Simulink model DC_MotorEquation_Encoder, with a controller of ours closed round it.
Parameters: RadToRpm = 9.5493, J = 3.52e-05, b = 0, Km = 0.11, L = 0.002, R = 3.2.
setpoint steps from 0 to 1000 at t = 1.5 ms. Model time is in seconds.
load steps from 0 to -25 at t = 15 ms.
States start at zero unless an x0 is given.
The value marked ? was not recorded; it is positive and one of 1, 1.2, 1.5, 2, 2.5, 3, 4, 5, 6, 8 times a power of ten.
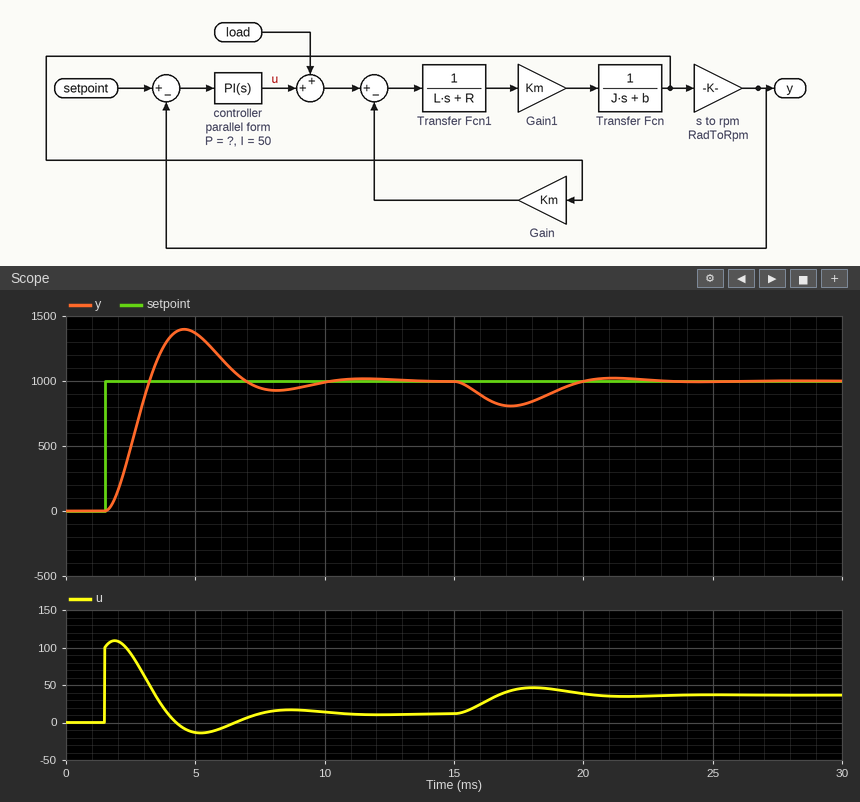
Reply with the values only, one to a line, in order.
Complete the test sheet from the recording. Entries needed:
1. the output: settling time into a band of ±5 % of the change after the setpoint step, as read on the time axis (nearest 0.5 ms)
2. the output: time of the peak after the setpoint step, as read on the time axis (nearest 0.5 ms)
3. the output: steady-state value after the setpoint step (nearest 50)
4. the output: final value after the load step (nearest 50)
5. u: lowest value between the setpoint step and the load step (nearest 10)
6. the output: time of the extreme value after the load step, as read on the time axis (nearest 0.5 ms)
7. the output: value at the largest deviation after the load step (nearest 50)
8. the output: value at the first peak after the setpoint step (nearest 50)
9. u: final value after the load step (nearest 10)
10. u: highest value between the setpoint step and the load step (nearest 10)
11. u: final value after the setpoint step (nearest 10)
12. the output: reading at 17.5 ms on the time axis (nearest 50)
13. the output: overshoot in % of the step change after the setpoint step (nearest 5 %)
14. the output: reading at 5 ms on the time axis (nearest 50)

9.0 ms
4.5 ms
1000
1000
-10
17.0 ms
800
1400
40
110
10
800
40 %
1350
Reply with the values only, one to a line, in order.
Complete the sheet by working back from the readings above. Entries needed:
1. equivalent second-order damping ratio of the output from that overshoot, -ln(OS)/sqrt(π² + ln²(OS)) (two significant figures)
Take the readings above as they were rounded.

0.28
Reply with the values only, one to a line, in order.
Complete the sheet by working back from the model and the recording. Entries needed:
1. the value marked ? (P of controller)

0.1
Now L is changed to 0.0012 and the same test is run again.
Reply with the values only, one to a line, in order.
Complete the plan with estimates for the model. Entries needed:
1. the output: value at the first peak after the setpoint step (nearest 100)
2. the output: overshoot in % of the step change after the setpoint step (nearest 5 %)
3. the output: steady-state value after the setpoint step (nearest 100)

1300
25 %
1000
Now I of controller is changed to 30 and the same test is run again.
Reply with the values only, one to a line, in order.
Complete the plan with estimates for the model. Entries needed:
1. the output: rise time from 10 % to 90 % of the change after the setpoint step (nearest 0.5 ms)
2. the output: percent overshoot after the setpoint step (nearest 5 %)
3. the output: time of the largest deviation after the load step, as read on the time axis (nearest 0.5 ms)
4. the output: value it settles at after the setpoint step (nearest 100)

1.5 ms
25 %
17.5 ms
1000
